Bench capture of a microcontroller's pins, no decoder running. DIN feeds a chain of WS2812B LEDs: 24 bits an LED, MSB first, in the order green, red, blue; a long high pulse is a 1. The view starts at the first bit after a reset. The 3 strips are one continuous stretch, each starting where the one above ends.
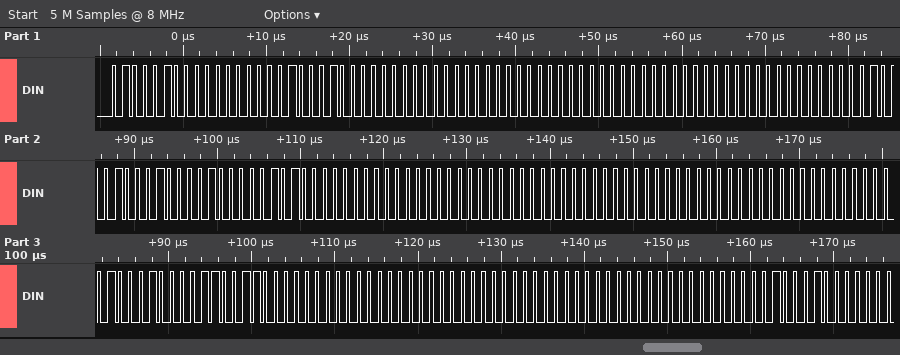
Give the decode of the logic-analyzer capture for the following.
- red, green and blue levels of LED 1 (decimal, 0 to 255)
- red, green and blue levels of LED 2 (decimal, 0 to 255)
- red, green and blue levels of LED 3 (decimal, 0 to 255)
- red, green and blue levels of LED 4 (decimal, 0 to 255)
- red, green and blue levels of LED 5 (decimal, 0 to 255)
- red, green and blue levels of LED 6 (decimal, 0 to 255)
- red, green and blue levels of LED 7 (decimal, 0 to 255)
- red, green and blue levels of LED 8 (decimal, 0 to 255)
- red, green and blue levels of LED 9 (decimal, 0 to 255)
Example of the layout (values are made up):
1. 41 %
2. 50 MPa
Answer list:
1. 0, 68, 68
2. 0, 0, 0
3. 0, 0, 0
4. 66, 68, 10
5. 0, 0, 0
6. 0, 0, 0
7. 68, 0, 51
8. 0, 0, 0
9. 0, 0, 0
